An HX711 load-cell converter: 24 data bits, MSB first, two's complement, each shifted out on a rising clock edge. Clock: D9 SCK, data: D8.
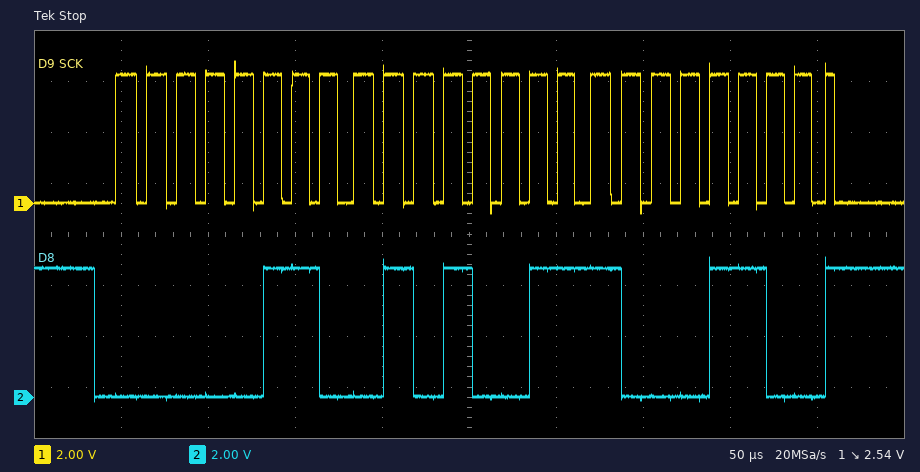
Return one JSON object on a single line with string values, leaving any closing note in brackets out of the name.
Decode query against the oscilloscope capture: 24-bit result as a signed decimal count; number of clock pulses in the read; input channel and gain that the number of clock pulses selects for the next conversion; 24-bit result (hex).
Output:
{"24-bit result as a signed decimal count": "414604", "number of clock pulses in the read": "25", "input channel and gain that the number of clock pulses selects for the next conversion": "channel A, gain 128", "24-bit result": "0x06538C"}
